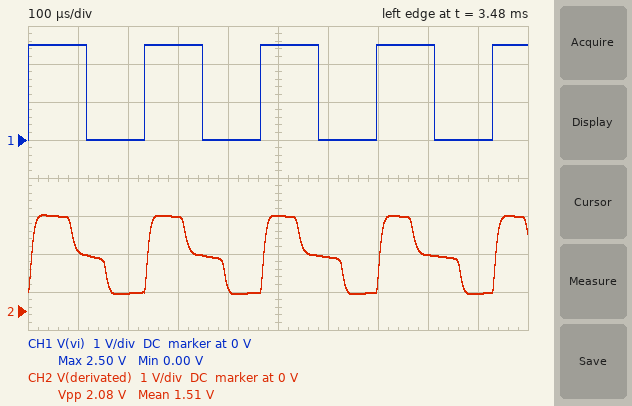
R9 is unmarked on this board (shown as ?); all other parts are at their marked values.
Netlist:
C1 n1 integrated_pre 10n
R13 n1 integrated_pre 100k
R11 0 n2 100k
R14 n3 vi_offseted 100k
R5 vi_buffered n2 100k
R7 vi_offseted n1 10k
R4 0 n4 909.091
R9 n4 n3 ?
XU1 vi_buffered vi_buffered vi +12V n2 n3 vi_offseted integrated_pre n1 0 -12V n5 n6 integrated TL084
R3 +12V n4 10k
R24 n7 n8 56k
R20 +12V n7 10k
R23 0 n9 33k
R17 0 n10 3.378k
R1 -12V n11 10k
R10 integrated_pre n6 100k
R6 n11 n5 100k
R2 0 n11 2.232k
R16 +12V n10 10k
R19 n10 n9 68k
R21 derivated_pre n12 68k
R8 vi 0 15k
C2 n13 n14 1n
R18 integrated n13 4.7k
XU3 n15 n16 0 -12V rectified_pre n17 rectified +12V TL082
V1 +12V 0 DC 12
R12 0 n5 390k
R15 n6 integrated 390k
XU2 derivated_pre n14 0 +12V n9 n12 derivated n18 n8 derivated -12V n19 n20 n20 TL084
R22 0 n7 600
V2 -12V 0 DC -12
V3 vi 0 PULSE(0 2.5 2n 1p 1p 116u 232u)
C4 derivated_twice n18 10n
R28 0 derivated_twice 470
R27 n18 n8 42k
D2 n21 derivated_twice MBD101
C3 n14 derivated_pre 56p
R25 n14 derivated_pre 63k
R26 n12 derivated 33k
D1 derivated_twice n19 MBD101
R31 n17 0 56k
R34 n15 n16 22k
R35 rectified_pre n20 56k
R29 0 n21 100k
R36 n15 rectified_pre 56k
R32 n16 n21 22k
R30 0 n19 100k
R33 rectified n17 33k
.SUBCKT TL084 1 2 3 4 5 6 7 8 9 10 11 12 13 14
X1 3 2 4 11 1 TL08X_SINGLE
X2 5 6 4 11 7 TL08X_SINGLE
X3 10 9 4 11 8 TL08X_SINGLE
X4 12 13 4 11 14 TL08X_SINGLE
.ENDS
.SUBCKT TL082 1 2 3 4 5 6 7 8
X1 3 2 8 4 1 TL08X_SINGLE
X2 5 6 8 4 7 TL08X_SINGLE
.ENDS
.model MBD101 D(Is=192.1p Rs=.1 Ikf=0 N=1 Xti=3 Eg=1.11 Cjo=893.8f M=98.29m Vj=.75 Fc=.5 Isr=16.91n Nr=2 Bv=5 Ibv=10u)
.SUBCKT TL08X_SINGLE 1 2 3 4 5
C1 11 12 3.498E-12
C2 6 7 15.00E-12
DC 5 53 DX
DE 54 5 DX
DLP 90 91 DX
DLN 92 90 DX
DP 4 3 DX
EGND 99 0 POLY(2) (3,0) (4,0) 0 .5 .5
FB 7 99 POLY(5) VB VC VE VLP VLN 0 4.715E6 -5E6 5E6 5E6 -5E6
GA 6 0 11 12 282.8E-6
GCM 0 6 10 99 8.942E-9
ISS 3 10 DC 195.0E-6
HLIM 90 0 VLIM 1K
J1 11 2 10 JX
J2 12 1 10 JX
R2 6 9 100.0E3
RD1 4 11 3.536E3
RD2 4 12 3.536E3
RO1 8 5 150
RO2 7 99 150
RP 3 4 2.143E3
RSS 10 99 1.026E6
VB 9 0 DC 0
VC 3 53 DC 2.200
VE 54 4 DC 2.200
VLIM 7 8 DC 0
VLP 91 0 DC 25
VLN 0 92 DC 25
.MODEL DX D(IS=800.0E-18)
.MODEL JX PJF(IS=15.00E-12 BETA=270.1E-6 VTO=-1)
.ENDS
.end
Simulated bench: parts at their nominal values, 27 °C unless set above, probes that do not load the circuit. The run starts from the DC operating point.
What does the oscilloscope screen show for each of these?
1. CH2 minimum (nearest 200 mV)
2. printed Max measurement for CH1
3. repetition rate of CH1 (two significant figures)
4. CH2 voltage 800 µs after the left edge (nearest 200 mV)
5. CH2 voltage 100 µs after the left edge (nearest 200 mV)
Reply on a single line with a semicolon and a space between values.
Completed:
400 mV; 2.50 V; 4.3 kHz; 1.4 V; 1.6 V
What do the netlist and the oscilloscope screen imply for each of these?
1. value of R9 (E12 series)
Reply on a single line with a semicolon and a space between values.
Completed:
270 kΩ
